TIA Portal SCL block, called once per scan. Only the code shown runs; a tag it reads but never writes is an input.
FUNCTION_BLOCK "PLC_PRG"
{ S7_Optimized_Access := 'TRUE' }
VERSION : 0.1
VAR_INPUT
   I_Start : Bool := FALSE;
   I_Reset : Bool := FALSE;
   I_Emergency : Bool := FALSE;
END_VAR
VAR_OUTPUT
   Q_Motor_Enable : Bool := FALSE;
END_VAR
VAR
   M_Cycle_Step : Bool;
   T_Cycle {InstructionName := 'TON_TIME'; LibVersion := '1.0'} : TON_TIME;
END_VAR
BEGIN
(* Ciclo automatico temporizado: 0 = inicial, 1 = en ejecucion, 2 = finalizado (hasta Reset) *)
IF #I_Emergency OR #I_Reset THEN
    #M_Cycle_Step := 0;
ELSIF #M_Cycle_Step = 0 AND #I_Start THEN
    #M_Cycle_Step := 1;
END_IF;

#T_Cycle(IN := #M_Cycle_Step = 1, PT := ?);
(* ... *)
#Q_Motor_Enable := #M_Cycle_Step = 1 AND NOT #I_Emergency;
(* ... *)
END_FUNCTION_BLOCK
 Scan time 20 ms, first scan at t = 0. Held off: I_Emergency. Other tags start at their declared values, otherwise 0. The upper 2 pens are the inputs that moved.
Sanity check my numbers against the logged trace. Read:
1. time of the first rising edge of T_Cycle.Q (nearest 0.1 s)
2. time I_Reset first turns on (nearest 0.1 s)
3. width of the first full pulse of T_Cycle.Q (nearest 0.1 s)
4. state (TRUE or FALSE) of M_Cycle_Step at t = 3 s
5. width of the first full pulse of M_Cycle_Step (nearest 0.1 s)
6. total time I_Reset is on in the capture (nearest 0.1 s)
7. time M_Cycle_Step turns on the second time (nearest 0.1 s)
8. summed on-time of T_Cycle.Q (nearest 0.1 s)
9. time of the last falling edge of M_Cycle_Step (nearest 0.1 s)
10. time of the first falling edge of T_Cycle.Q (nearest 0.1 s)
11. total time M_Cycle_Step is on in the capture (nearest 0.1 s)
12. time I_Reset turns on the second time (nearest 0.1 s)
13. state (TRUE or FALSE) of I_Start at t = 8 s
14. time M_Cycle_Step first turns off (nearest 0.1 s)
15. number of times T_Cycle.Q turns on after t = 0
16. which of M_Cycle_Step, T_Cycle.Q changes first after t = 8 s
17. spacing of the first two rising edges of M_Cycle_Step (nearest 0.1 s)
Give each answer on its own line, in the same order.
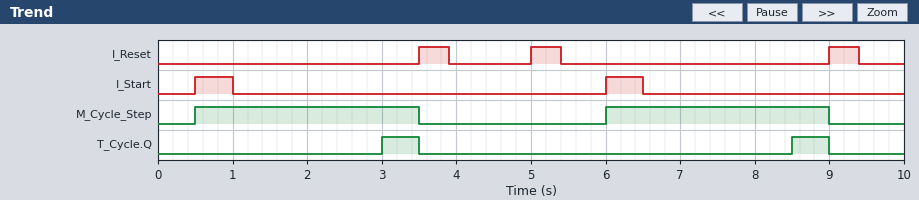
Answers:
3.0 s
3.5 s
0.5 s
TRUE
3.0 s
1.2 s
6.0 s
1.0 s
9.0 s
3.5 s
6.0 s
5.0 s
FALSE
3.5 s
2
T_Cycle.Q
5.5 s
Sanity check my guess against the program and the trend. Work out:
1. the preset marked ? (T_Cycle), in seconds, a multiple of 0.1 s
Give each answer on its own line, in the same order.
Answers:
2.5 s
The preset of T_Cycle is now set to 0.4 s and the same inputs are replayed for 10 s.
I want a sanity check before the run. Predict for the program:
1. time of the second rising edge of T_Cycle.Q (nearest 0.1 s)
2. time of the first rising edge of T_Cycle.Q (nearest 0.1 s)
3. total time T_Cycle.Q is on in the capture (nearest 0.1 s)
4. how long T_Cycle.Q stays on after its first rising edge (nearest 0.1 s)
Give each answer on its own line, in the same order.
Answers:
6.4 s
0.9 s
5.2 s
2.6 s
